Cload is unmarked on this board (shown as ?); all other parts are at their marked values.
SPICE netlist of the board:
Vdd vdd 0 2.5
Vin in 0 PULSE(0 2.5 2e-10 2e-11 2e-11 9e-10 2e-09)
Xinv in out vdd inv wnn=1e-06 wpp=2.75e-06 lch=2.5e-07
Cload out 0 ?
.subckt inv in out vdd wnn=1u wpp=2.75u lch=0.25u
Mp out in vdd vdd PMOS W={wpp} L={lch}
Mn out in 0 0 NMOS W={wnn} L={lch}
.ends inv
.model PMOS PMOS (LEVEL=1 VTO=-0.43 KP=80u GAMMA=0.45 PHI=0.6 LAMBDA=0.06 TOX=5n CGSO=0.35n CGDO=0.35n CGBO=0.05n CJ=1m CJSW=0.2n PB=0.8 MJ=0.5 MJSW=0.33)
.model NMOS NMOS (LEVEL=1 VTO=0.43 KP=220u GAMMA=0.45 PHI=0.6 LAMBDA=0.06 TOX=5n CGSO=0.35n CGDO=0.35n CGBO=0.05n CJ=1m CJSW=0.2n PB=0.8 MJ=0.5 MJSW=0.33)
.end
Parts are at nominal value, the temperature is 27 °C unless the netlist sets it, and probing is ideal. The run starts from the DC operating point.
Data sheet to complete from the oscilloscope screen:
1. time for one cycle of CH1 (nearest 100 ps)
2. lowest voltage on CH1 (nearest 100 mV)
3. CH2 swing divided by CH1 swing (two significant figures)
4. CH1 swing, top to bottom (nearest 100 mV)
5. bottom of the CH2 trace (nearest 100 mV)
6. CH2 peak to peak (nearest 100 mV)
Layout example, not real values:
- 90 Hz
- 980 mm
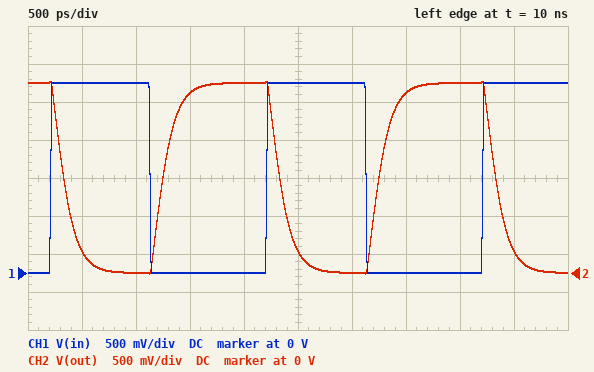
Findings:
- 2.0 ns
- 0 V
- 1.0
- 2.5 V
- 0 V
- 2.5 V
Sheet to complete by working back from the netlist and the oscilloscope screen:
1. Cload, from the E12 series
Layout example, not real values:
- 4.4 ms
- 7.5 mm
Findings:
- 180 fF
